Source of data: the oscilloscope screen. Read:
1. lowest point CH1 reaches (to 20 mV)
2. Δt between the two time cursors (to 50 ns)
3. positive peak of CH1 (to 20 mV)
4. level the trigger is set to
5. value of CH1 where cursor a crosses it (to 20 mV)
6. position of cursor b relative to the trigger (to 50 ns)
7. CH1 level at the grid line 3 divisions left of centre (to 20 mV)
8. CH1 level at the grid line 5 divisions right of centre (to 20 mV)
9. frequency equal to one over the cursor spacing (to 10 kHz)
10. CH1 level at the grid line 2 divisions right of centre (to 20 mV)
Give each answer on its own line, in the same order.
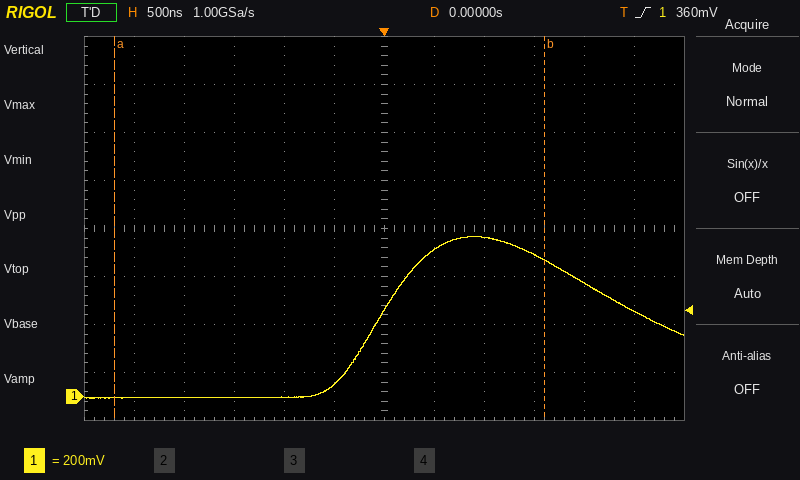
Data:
0 mV
4.30 µs
660 mV
360 mV
0 mV
+1.60 µs
0 mV
360 mV
230 kHz
660 mV
